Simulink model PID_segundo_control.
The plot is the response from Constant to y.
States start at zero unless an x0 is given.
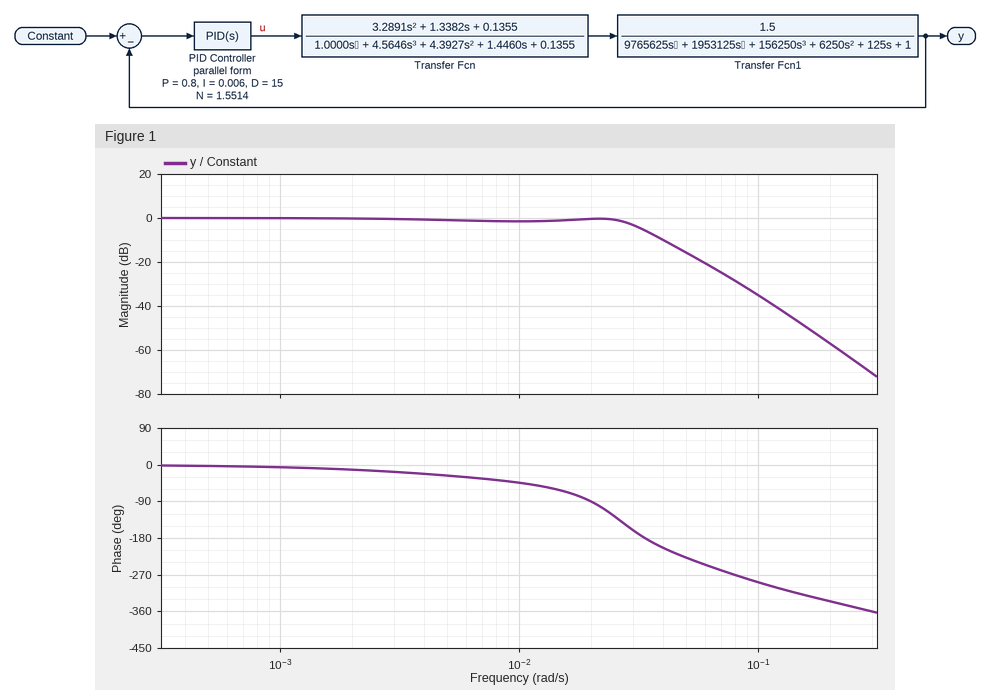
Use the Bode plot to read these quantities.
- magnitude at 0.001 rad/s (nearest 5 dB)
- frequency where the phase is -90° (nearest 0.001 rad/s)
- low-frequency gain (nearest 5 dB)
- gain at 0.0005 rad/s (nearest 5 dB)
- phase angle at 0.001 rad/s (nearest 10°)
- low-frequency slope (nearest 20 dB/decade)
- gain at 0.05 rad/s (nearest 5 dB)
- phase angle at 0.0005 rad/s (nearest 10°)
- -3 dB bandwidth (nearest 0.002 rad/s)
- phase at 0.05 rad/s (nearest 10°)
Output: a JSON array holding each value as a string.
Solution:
["0 dB", "0.020 rad/s", "0 dB", "0 dB", "-10°", "0 dB/decade", "-15 dB", "0°", "0.030 rad/s", "-230°"]
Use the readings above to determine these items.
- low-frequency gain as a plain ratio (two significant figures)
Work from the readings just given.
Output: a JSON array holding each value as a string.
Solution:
["1.0"]
